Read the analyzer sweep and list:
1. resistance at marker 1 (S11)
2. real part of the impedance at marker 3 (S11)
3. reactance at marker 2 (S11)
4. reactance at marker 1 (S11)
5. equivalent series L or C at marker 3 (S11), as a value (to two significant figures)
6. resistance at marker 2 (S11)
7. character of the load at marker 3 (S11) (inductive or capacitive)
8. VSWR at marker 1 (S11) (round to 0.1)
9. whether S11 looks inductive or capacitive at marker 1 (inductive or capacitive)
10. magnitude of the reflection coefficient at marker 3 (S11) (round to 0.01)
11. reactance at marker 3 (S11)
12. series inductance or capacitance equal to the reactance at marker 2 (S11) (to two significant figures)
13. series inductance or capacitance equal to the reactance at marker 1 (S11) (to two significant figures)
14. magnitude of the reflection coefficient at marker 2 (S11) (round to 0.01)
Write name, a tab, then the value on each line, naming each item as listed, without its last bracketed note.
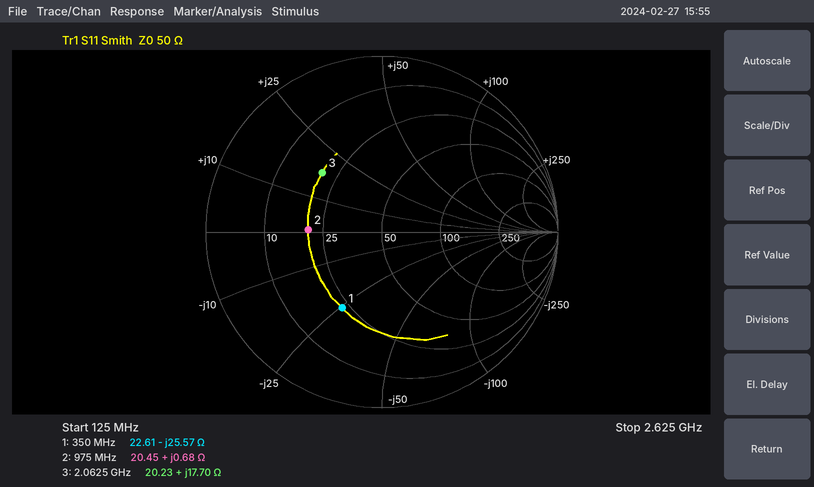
resistance at marker 1	22.61 Ω
real part of the impedance at marker 3	20.23 Ω
reactance at marker 2	+0.68 Ω
reactance at marker 1	-25.57 Ω
equivalent series L or C at marker 3 (S11), as a value	1.4 nH
resistance at marker 2	20.45 Ω
character of the load at marker 3 (S11)	inductive
VSWR at marker 1 (S11)	2.9
whether S11 looks inductive or capacitive at marker 1	capacitive
magnitude of the reflection coefficient at marker 3 (S11)	0.48
reactance at marker 3	+17.70 Ω
series inductance or capacitance equal to the reactance at marker 2 (S11)	110 pH
series inductance or capacitance equal to the reactance at marker 1 (S11)	18 pF
magnitude of the reflection coefficient at marker 2 (S11)	0.42
